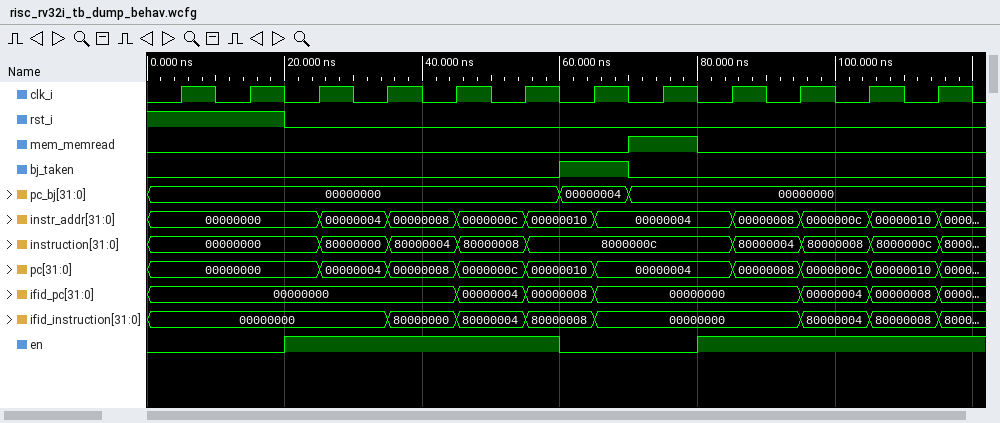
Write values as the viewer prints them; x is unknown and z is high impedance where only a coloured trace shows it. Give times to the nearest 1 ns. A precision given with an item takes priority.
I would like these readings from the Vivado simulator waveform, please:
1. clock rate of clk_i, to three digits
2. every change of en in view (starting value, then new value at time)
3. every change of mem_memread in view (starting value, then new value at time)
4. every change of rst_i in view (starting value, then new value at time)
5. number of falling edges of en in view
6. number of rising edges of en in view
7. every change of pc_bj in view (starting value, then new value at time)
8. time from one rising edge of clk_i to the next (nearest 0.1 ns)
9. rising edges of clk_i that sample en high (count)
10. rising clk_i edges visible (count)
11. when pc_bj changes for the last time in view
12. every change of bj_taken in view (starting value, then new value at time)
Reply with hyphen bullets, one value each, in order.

- 100 MHz
- 0, 1 at 20 ns, 0 at 60 ns, 1 at 80 ns
- 0, 1 at 70 ns, 0 at 80 ns
- 1, 0 at 20 ns
- 1
- 2
- 00000000, 00000004 at 60 ns, 00000000 at 70 ns
- 10 ns
- 8
- 12
- 70 ns
- 0, 1 at 60 ns, 0 at 70 ns
